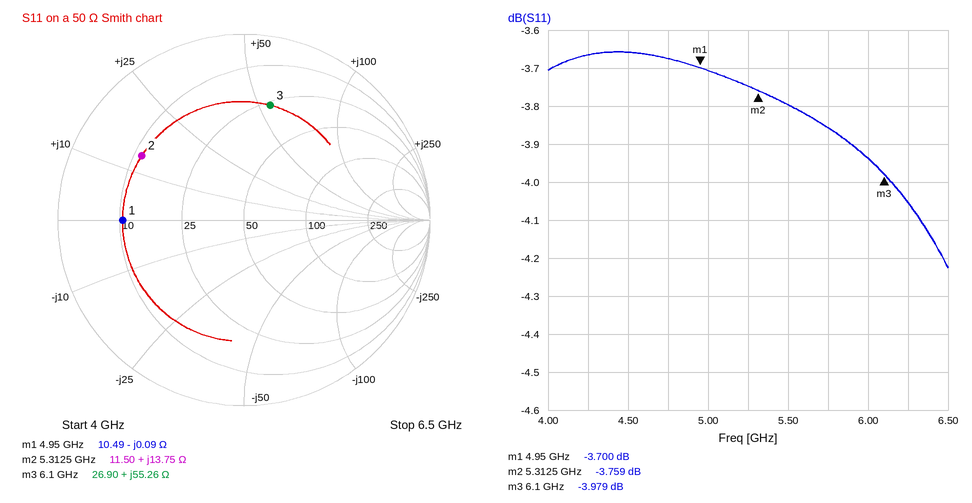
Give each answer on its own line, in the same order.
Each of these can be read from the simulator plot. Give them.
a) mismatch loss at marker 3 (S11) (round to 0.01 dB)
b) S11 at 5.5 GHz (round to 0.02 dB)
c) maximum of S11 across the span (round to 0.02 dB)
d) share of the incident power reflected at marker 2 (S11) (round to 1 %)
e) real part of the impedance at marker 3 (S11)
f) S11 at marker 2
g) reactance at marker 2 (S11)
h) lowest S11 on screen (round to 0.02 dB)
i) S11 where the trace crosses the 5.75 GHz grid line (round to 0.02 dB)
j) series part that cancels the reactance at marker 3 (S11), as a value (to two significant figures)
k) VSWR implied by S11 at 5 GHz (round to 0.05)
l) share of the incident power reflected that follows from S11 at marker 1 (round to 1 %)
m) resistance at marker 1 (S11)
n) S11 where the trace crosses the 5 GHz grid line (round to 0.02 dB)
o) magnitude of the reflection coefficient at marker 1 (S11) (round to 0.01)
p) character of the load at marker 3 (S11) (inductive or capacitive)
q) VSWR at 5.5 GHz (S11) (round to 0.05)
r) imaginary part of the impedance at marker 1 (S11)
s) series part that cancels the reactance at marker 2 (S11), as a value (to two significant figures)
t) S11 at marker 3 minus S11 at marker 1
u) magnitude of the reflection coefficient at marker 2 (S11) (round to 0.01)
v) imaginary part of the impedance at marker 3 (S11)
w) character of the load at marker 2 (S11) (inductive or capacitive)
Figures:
2.22 dB
-3.80 dB
-3.66 dB
42 %
26.90 Ω
-3.759 dB
+13.75 Ω
-4.22 dB
-3.86 dB
470 fF
4.75
43 %
10.49 Ω
-3.70 dB
0.65
inductive
4.65
-0.09 Ω
2.2 pF
-0.279 dB
0.65
+55.26 Ω
inductive
